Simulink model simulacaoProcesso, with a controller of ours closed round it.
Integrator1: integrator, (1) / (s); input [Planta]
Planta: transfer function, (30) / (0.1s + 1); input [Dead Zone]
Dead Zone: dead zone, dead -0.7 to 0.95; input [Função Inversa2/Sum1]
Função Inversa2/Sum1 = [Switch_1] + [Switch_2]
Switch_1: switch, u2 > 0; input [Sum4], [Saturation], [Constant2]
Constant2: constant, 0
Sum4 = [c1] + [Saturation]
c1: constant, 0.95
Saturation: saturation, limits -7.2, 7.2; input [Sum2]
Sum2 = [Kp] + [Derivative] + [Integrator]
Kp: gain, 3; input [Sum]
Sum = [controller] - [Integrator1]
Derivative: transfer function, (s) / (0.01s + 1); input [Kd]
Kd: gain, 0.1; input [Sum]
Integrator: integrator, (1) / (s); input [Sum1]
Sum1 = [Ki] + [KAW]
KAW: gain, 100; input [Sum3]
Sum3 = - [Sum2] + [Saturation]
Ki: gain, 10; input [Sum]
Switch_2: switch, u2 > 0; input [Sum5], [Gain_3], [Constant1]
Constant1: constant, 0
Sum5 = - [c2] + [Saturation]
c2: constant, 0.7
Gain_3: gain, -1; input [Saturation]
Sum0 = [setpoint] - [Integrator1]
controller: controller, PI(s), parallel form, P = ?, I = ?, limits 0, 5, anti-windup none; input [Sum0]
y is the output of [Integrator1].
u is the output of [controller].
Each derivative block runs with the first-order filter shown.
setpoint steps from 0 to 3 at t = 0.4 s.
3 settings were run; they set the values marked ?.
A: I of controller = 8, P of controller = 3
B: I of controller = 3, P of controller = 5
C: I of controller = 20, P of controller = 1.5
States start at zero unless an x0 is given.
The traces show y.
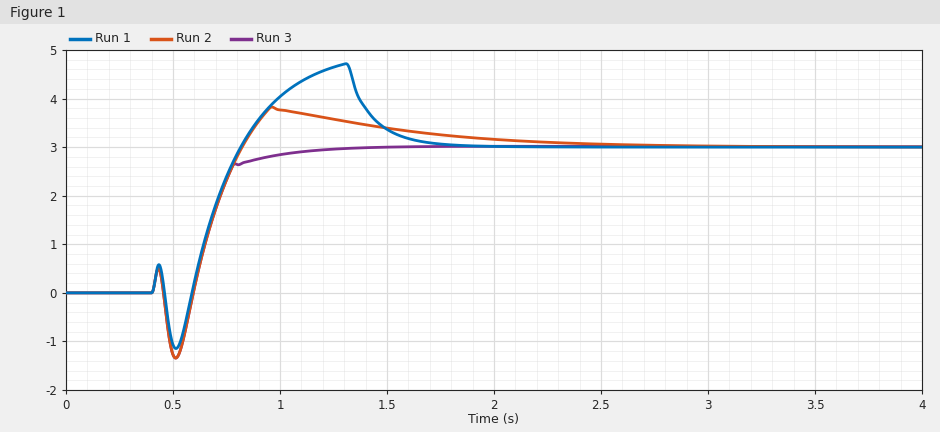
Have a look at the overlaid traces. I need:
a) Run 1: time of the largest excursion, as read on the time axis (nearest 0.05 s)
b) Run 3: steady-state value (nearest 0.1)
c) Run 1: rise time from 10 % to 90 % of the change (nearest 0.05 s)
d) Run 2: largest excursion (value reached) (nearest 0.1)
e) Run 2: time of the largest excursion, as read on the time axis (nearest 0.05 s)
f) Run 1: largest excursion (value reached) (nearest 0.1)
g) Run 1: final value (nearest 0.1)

1.30 s
3.0
0.35 s
3.8
0.95 s
4.7
3.0
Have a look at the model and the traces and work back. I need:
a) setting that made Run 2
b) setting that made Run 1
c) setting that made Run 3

A
C
B
